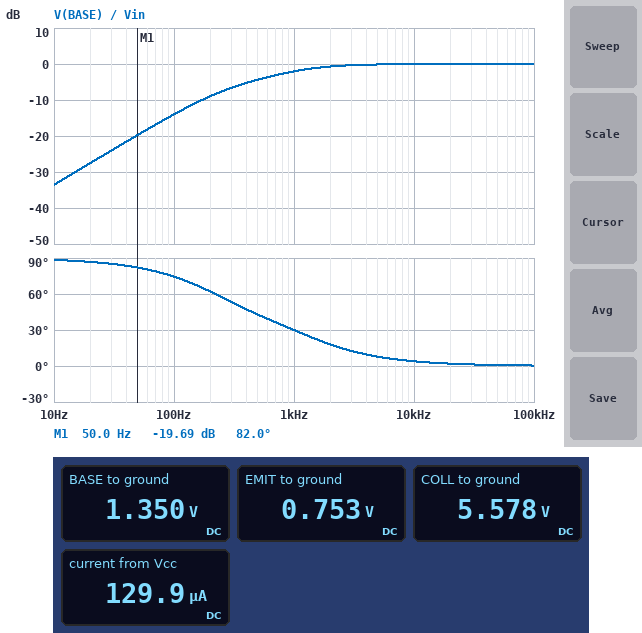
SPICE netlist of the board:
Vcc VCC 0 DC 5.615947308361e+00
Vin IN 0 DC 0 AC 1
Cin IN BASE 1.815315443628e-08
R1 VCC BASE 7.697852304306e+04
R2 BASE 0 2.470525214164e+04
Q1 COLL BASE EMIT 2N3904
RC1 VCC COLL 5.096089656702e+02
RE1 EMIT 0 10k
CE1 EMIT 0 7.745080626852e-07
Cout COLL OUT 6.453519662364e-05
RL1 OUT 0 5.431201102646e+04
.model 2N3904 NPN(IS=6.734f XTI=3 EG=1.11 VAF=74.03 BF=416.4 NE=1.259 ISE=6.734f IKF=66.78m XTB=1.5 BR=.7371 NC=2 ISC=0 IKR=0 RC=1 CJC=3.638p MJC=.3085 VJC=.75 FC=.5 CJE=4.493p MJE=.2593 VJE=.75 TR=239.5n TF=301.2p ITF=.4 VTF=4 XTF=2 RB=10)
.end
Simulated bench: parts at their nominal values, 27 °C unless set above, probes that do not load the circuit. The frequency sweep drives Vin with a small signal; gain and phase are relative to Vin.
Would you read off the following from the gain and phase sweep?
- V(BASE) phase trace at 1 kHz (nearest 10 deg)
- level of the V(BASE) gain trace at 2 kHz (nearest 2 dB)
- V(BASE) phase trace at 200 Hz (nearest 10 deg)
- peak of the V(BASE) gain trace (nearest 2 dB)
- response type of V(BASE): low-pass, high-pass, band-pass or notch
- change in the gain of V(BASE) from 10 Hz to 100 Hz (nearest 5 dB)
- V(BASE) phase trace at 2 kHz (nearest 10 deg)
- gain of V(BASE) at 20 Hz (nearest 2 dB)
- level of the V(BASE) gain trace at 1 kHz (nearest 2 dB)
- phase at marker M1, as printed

30 deg
0 dB
60 deg
0 dB
high-pass
20 dB
20 deg
-28 dB
-2 dB
82.0 deg
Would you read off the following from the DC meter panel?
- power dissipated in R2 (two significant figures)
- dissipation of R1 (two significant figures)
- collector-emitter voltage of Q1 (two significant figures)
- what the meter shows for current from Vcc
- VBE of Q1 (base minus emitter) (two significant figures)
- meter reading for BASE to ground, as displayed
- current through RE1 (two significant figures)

74 µW
240 µW
4.8 V
129.9 µA
600 mV
1.350 V
75 µA
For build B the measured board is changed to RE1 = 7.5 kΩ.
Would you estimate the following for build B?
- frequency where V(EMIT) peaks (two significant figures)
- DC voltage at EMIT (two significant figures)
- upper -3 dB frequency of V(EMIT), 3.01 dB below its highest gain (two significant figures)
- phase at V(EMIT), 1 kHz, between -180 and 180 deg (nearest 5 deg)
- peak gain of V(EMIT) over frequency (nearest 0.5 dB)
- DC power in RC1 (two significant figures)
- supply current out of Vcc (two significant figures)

620 Hz
740 mV
1.8 kHz
-20 deg
-6.0 dB
4.9 µW
150 µA
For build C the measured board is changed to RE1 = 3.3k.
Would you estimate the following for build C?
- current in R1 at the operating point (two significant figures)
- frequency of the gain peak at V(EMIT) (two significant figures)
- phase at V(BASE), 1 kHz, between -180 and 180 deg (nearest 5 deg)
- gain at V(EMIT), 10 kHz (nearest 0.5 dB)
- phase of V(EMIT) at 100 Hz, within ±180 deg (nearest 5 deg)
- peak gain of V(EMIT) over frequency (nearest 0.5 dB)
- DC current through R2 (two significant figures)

56 µA
920 Hz
25 deg
-15.5 dB
70 deg
-4.5 dB
54 µA
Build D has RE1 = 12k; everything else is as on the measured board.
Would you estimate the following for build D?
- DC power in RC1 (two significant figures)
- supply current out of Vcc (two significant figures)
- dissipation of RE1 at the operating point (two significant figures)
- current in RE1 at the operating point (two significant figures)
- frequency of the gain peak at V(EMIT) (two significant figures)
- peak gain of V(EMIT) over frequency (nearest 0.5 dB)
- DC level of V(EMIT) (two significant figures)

2.0 µW
120 µA
48 µW
63 µA
500 Hz
-7.5 dB
760 mV
